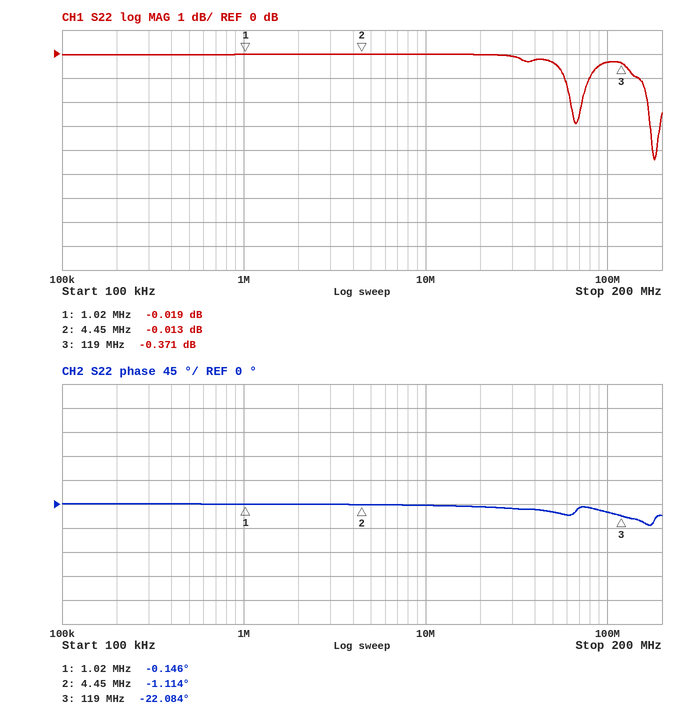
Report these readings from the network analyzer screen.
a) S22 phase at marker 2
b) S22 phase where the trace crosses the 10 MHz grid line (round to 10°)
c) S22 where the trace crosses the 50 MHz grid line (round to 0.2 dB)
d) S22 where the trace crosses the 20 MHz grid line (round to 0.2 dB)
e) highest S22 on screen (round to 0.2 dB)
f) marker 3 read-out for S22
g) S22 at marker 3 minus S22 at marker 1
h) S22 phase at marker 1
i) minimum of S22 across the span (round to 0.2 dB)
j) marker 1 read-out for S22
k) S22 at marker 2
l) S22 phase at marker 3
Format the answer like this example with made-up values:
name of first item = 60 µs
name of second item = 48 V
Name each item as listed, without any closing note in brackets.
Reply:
S22 phase at marker 2 = -1.114°
S22 phase where the trace crosses the 10 MHz grid line = 0°
S22 where the trace crosses the 50 MHz grid line = -0.4 dB
S22 where the trace crosses the 20 MHz grid line = 0.0 dB
highest S22 on screen = 0.0 dB
marker 3 read-out for S22 = -0.371 dB
S22 at marker 3 minus S22 at marker 1 = -0.352 dB
S22 phase at marker 1 = -0.146°
minimum of S22 across the span = -4.4 dB
marker 1 read-out for S22 = -0.019 dB
S22 at marker 2 = -0.013 dB
S22 phase at marker 3 = -22.084°
